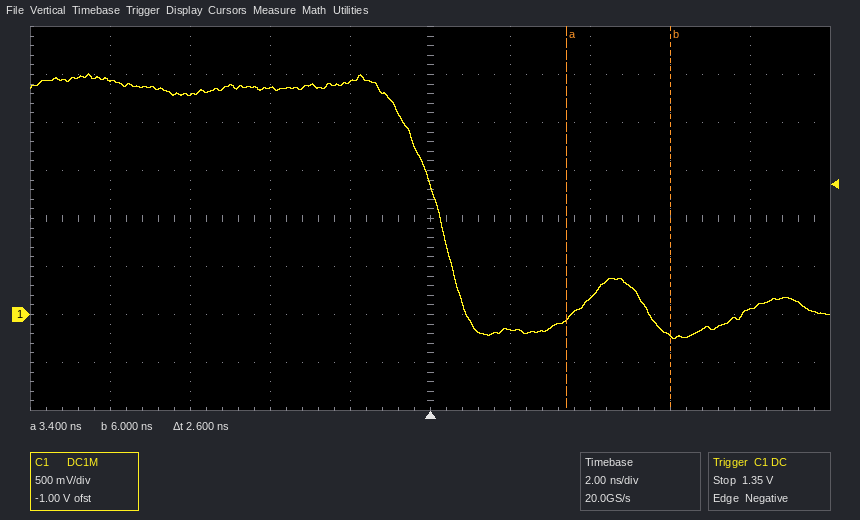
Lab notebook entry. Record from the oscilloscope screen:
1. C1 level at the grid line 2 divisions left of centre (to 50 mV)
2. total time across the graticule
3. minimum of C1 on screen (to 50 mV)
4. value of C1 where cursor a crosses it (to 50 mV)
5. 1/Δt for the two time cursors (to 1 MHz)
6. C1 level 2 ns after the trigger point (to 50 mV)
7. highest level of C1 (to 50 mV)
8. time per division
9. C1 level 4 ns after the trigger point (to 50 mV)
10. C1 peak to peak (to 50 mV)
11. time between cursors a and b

2.35 V
20 ns
-250 mV
-50 mV
385 MHz
-150 mV
2.50 V
2 ns
150 mV
2.75 V
2.6 ns
